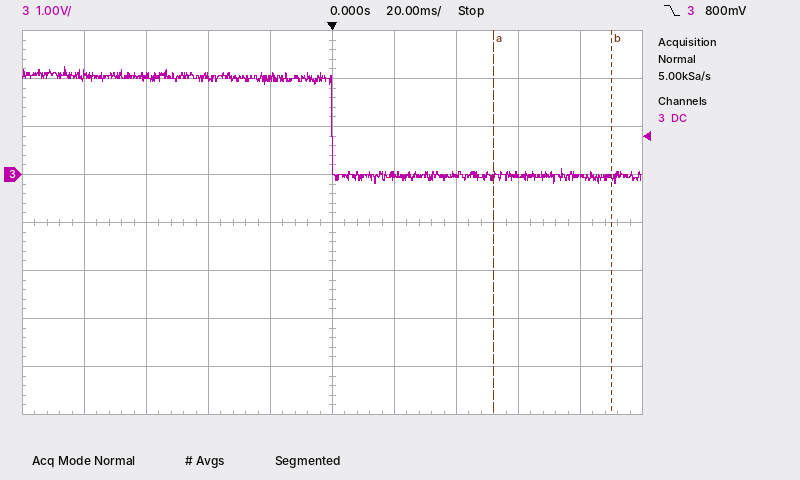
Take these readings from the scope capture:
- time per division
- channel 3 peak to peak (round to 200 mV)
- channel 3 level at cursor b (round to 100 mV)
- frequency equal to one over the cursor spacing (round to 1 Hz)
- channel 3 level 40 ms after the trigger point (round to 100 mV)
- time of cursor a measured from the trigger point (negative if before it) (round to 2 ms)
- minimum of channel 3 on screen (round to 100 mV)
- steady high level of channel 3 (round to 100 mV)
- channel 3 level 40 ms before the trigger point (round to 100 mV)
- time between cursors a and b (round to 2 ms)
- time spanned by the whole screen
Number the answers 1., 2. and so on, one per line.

1. 20 ms
2. 2.4 V
3. -100 mV
4. 26 Hz
5. 0.0 V
6. +52 ms
7. -200 mV
8. 2.0 V
9. 2.0 V
10. 38 ms
11. 200 ms
